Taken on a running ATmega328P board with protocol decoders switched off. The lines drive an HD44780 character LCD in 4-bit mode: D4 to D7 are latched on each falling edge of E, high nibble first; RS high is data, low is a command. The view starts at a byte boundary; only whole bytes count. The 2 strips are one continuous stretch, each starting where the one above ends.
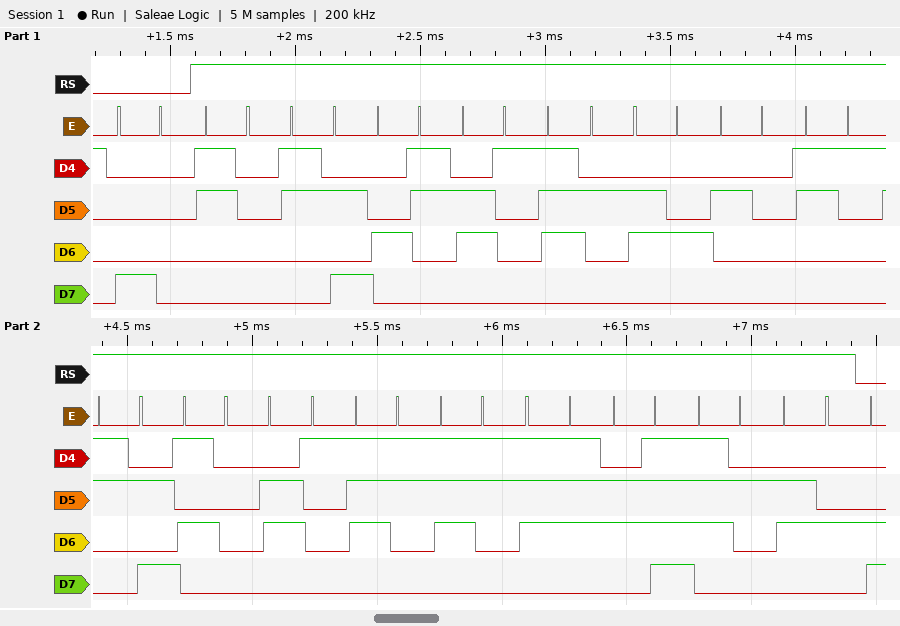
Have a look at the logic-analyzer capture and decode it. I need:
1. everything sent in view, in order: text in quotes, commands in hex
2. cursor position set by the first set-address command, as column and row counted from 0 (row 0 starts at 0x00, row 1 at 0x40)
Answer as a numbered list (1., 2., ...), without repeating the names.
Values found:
1. 0x80 "0:Card 1:Password"
2. column 0, row 0
